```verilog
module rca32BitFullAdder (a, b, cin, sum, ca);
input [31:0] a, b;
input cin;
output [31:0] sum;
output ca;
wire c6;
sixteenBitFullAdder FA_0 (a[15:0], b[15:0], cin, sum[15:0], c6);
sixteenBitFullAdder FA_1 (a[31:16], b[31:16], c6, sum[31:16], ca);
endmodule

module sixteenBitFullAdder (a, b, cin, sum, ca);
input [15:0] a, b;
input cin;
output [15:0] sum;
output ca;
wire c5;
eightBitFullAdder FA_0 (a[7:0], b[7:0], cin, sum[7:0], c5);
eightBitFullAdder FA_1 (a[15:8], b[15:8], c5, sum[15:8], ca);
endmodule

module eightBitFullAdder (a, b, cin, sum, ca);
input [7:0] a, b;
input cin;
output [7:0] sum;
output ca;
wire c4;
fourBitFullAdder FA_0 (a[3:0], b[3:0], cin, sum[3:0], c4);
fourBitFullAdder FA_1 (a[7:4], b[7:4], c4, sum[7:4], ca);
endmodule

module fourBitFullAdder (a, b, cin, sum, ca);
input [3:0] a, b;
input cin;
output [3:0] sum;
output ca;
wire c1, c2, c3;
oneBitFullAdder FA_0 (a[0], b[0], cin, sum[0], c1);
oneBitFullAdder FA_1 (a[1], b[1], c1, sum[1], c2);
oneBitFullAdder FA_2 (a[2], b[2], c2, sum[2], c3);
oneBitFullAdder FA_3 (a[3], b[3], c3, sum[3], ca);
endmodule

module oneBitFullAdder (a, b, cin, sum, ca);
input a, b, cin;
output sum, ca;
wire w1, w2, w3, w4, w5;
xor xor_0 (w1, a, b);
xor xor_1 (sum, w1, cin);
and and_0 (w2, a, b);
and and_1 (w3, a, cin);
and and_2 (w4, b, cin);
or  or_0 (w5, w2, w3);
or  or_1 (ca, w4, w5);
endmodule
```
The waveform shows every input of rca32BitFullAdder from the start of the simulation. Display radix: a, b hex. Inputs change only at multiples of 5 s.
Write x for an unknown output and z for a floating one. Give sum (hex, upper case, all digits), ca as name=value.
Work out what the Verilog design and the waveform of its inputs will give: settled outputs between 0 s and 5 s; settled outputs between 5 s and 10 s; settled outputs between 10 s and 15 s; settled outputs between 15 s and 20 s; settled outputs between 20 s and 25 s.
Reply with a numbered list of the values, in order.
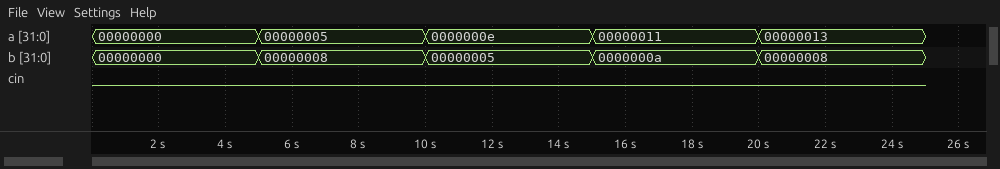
1. sum=00000000, ca=0
2. sum=0000000D, ca=0
3. sum=00000013, ca=0
4. sum=0000001B, ca=0
5. sum=0000001B, ca=0
